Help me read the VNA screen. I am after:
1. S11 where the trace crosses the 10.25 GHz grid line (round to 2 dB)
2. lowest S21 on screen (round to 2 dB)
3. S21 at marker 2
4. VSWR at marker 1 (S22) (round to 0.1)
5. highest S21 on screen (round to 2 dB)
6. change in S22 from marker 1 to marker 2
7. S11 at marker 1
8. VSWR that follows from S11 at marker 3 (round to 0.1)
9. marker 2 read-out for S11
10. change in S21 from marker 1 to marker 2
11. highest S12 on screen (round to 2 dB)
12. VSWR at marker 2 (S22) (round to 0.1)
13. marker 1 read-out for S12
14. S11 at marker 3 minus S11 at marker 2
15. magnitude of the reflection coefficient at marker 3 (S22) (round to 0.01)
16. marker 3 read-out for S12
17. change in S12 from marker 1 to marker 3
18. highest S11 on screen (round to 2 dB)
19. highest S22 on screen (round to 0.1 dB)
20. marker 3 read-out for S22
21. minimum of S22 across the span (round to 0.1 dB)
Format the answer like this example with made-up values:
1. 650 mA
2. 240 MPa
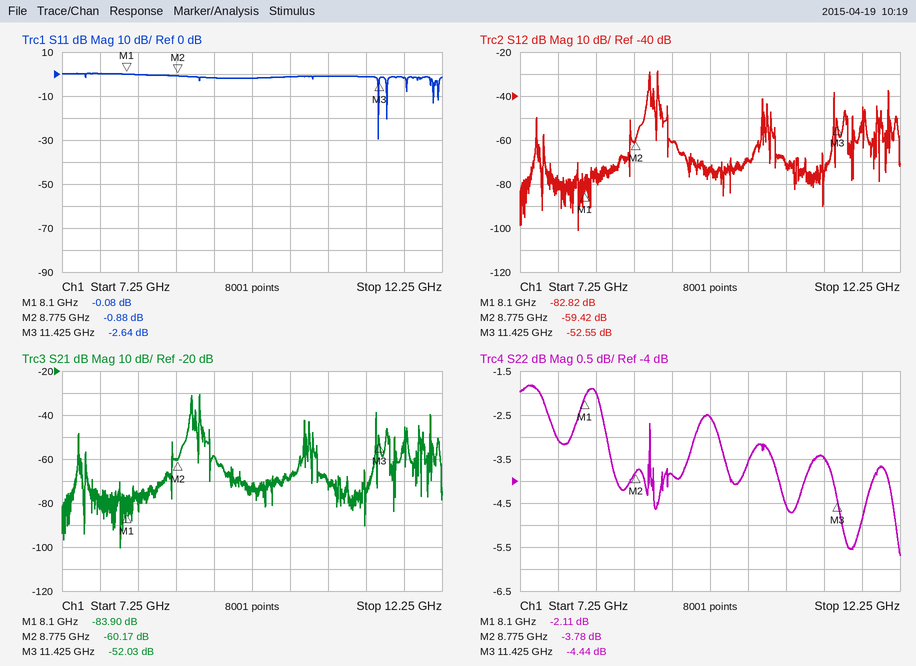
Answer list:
1. -2 dB
2. -100 dB
3. -60.17 dB
4. 8.3
5. -30 dB
6. -1.67 dB
7. -0.08 dB
8. 6.6
9. -0.88 dB
10. 23.73 dB
11. -28 dB
12. 4.7
13. -82.82 dB
14. -1.76 dB
15. 0.60
16. -52.55 dB
17. 30.27 dB
18. 0 dB
19. -1.8 dB
20. -4.44 dB
21. -5.7 dB
